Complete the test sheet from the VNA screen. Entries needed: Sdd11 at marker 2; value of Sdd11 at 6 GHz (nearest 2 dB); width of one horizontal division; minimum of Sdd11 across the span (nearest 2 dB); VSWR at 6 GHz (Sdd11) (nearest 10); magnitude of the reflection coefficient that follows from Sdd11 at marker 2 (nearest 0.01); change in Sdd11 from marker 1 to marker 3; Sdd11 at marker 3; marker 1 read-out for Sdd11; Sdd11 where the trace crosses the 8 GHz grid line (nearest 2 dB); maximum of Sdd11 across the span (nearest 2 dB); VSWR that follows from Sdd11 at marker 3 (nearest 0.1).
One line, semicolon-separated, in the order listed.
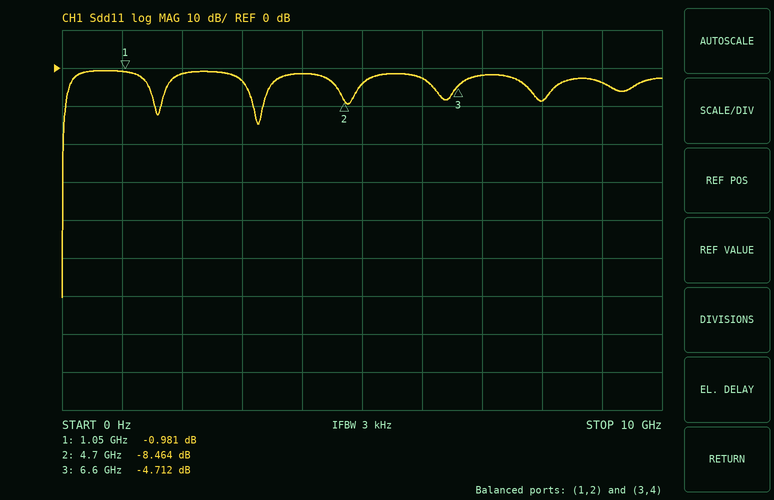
-8.464 dB; -2 dB; 1 GHz; -60 dB; 10; 0.38; -3.731 dB; -4.712 dB; -0.981 dB; -8 dB; 0 dB; 3.8
